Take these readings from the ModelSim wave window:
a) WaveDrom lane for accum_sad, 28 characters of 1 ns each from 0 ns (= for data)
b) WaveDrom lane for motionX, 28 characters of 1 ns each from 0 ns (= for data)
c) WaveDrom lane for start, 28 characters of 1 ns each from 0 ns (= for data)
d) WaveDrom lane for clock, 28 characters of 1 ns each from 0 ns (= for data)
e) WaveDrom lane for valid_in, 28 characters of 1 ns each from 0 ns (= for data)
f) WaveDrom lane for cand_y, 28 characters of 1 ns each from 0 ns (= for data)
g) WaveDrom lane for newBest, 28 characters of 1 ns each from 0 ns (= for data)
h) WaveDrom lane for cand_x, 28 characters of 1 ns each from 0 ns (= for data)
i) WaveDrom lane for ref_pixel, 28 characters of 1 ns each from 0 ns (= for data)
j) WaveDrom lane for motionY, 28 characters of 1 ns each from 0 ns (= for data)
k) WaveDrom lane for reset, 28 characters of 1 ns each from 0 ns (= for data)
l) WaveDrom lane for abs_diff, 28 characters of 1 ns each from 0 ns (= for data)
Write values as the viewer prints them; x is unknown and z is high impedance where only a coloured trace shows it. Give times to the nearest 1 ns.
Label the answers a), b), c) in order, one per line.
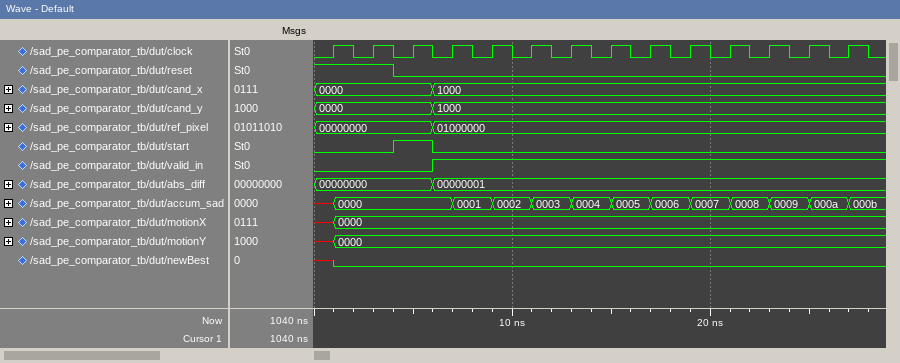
a) {name: 'accum_sad', wave: 'x=.....=.=.=.=.=.=.=.=.=.=.=', data: '0000 0001 0002 0003 0004 0005 0006 0007 0008 0009 000a 000b'}
b) {name: 'motionX', wave: 'x=..........................', data: '0000'}
c) {name: 'start', wave: '0...1.0.....................'}
d) {name: 'clock', wave: '0101010101010101010101010101'}
e) {name: 'valid_in', wave: '0.....1.....................'}
f) {name: 'cand_y', wave: '=.....=.....................', data: '0000 1000'}
g) {name: 'newBest', wave: 'x0..........................'}
h) {name: 'cand_x', wave: '=.....=.....................', data: '0000 1000'}
i) {name: 'ref_pixel', wave: '=.....=.....................', data: '00000000 01000000'}
j) {name: 'motionY', wave: 'x=..........................', data: '0000'}
k) {name: 'reset', wave: '1...0.......................'}
l) {name: 'abs_diff', wave: '=.....=.....................', data: '00000000 00000001'}
